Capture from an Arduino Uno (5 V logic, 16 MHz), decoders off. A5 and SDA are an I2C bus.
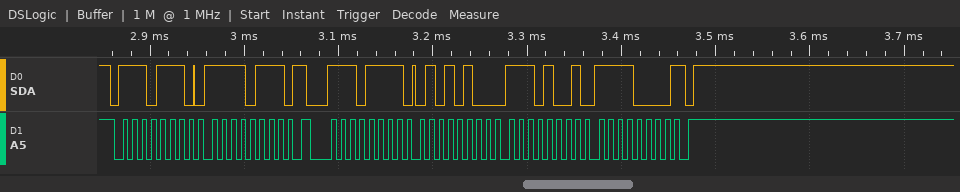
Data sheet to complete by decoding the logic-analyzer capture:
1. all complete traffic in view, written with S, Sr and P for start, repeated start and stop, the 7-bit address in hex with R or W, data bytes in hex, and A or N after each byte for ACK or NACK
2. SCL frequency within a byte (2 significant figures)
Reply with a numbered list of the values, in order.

1. S 77W A F7 A Sr 77R A 54 A E9 A F0 N P
2. 100 kHz
